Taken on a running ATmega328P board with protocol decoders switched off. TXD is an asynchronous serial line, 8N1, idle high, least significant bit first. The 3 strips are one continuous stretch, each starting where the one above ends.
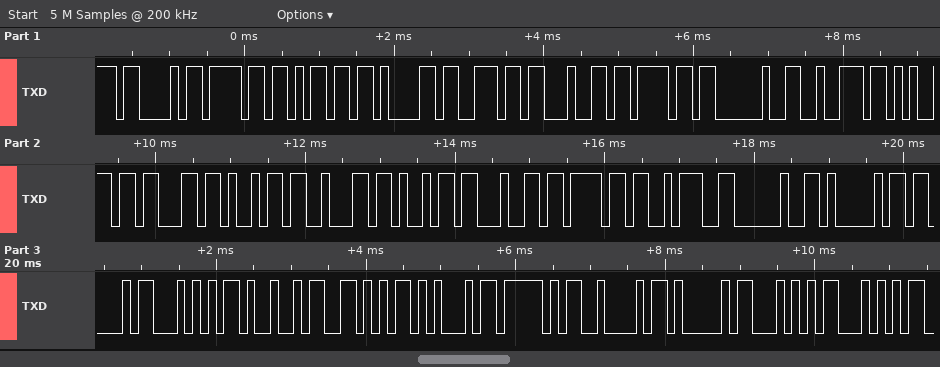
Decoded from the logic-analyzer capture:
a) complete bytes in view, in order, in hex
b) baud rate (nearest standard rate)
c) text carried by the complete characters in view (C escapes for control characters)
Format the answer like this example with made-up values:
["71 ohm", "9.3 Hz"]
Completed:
["43 6F 6D 61 6E 64 6F 20 72 65 63 69 62 69 64 6F 3A 20 41 43 54 49 56 45 5F 42 41 54 54", "9600 baud", "\"Comando recibido: ACTIVE_BATT\""]
